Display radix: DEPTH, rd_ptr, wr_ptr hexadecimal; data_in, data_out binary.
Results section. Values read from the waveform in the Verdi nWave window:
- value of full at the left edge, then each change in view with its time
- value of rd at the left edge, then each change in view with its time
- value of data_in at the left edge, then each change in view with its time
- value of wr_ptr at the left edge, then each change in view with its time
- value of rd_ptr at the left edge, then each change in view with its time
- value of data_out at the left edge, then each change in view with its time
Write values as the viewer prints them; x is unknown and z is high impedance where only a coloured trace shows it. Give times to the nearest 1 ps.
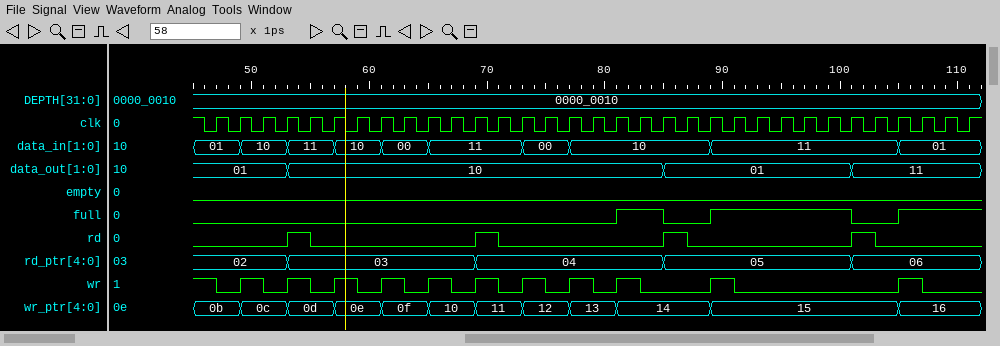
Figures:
0, 1 at 81 ps, 0 at 85 ps, 1 at 89 ps, 0 at 101 ps, 1 at 105 ps
0, 1 at 53 ps, 0 at 55 ps, 1 at 69 ps, 0 at 71 ps, 1 at 85 ps, 0 at 87 ps, 1 at 101 ps, 0 at 103 ps
01, 10 at 49 ps, 11 at 53 ps, 10 at 57 ps, 00 at 61 ps, 11 at 65 ps, 00 at 73 ps, 10 at 77 ps, 11 at 89 ps, 01 at 105 ps
0b, 0c at 49 ps, 0d at 53 ps, 0e at 57 ps, 0f at 61 ps, 10 at 65 ps, 11 at 69 ps, 12 at 73 ps, 13 at 77 ps, 14 at 81 ps, 15 at 89 ps, 16 at 105 ps
02, 03 at 53 ps, 04 at 69 ps, 05 at 85 ps, 06 at 101 ps
01, 10 at 53 ps, 01 at 85 ps, 11 at 101 ps
